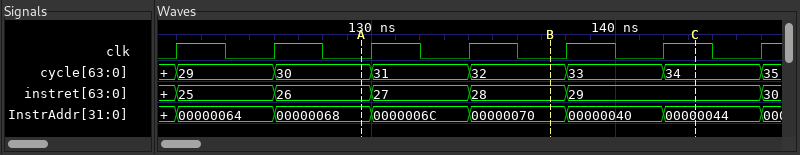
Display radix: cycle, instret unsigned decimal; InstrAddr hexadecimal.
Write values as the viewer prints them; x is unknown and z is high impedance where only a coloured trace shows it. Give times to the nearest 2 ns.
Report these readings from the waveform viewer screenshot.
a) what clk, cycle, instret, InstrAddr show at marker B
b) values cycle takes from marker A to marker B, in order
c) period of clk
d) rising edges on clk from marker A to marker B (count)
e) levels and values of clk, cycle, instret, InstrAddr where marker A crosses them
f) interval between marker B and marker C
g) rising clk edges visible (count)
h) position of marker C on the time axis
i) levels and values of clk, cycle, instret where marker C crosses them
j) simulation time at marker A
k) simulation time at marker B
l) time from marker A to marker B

clk=0, cycle=32, instret=28, InstrAddr=00000070
30, 31, 32
4 ns
2
clk=0, cycle=30, instret=26, InstrAddr=00000068
6 ns
7
144 ns
clk=1, cycle=34, instret=29
130 ns
138 ns
8 ns
